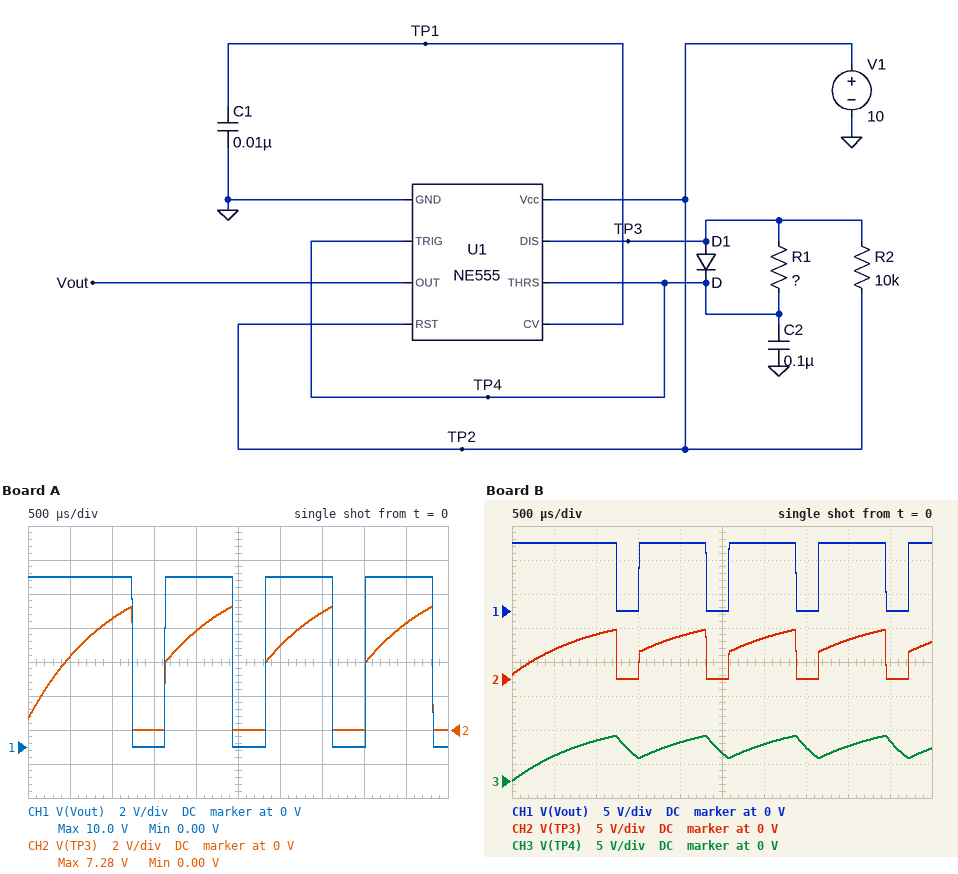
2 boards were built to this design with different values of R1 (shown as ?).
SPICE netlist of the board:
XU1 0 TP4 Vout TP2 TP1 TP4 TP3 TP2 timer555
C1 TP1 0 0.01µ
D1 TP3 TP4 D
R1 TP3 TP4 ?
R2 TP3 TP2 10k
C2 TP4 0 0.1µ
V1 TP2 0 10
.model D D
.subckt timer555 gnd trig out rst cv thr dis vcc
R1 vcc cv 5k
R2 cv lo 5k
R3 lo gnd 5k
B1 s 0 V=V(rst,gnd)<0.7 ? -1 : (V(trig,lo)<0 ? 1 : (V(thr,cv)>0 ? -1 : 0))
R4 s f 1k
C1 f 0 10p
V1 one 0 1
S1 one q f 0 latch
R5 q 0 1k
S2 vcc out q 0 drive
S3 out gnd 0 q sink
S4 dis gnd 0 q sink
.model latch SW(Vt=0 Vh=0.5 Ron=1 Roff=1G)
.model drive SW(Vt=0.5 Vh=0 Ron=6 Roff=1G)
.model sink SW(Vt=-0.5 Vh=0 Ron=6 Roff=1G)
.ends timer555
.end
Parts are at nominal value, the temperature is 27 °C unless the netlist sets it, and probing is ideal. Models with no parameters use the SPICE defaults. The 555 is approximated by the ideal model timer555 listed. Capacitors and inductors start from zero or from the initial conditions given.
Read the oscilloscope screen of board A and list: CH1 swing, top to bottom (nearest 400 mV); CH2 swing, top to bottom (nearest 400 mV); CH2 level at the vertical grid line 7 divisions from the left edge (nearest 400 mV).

10.0 V
7.2 V
6.8 V
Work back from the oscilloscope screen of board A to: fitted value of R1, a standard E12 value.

5.6 kΩ
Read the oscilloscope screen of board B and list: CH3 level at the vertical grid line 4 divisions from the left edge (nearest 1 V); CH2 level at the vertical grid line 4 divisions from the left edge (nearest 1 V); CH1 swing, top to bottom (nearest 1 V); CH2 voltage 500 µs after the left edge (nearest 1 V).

6 V
6 V
10 V
4 V
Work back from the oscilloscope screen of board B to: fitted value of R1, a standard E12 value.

3.9 kΩ
